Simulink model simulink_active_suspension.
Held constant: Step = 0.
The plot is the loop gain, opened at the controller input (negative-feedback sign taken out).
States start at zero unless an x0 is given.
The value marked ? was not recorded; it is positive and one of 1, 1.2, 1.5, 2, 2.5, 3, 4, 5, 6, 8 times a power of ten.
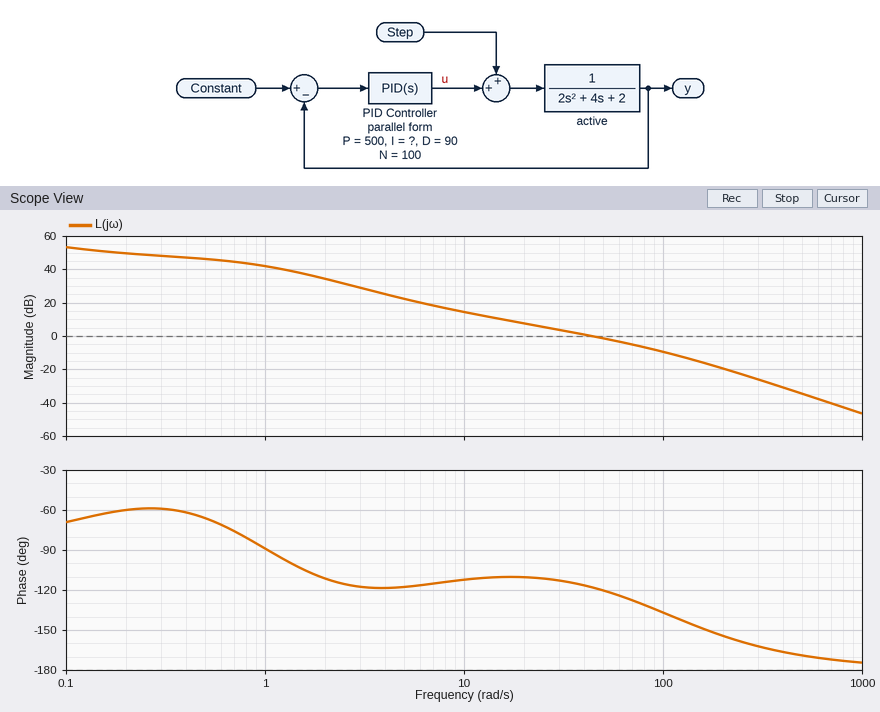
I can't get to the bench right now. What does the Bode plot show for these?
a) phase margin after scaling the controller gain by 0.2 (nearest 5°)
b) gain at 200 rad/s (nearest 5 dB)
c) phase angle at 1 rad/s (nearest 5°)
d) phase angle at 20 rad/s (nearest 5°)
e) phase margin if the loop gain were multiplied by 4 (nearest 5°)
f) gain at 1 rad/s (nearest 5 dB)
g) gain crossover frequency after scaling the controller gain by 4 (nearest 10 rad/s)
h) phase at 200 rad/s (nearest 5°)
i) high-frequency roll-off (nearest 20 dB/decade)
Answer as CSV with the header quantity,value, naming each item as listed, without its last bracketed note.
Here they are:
quantity,value
phase margin after scaling the controller gain by 0.2,70°
gain at 200 rad/s,-20 dB
phase angle at 1 rad/s,-90°
phase angle at 20 rad/s,-110°
phase margin if the loop gain were multiplied by 4,40°
gain at 1 rad/s,40 dB
gain crossover frequency after scaling the controller gain by 4,120 rad/s
phase at 200 rad/s,-155°
high-frequency roll-off,-40 dB/decade
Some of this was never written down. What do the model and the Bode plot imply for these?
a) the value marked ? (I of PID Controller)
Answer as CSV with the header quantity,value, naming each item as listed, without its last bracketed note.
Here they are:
quantity,value
the value marked ?,80
